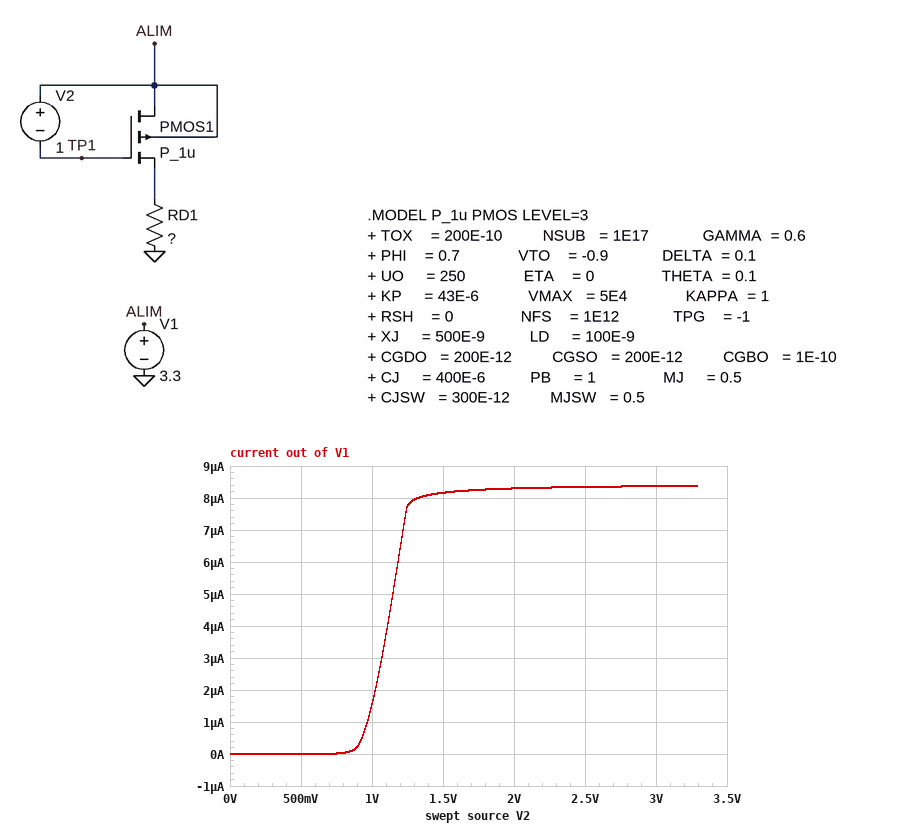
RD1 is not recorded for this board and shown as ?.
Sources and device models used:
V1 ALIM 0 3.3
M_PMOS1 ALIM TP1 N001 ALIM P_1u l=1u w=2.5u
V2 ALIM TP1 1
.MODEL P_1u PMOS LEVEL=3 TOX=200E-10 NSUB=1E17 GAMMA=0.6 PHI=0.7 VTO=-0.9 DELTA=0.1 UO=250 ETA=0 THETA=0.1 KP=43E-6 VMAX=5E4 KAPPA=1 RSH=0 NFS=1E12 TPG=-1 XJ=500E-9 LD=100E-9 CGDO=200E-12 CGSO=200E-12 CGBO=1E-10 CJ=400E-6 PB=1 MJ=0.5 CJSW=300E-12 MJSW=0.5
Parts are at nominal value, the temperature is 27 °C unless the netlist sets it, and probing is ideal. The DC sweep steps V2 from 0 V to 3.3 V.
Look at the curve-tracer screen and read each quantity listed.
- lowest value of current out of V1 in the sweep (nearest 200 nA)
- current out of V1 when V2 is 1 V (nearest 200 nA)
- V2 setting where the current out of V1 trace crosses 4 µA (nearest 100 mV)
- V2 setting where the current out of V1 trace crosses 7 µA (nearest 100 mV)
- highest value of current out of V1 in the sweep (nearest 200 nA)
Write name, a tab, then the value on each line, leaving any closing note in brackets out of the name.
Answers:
lowest value of current out of V1 in the sweep	0 A
current out of V1 when V2 is 1 V	1.6 µA
V2 setting where the current out of V1 trace crosses 4 µA	1.1 V
V2 setting where the current out of V1 trace crosses 7 µA	1.2 V
highest value of current out of V1 in the sweep	8.4 µA
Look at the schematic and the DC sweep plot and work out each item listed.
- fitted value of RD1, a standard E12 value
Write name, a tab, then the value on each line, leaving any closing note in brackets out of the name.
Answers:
fitted value of RD1, a standard E12 value	390 kΩ
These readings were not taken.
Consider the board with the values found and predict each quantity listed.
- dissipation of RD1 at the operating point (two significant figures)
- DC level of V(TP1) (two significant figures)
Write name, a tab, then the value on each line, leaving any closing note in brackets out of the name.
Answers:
dissipation of RD1 at the operating point	940 nW
DC level of V(TP1)	2.3 V
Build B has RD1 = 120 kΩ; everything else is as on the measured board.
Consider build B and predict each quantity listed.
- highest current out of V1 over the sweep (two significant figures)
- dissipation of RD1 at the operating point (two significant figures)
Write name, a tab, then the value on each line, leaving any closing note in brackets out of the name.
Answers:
highest current out of V1 over the sweep	27 µA
dissipation of RD1 at the operating point	300 nW
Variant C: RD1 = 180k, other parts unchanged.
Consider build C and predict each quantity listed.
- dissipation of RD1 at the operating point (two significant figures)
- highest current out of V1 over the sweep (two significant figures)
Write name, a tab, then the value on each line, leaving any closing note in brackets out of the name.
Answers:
dissipation of RD1 at the operating point	440 nW
highest current out of V1 over the sweep	18 µA
